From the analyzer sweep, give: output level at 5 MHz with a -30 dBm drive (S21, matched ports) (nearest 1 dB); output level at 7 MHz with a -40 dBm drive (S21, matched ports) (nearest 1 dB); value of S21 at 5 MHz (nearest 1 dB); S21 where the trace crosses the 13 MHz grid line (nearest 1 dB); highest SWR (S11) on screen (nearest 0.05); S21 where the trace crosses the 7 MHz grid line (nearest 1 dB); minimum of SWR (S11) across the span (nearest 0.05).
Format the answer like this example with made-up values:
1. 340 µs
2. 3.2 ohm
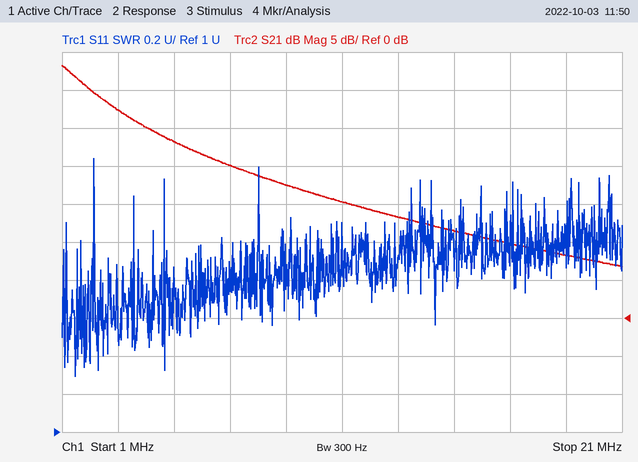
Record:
1. -7 dBm
2. -20 dBm
3. 23 dB
4. 13 dB
5. 2.45
6. 20 dB
7. 1.30
